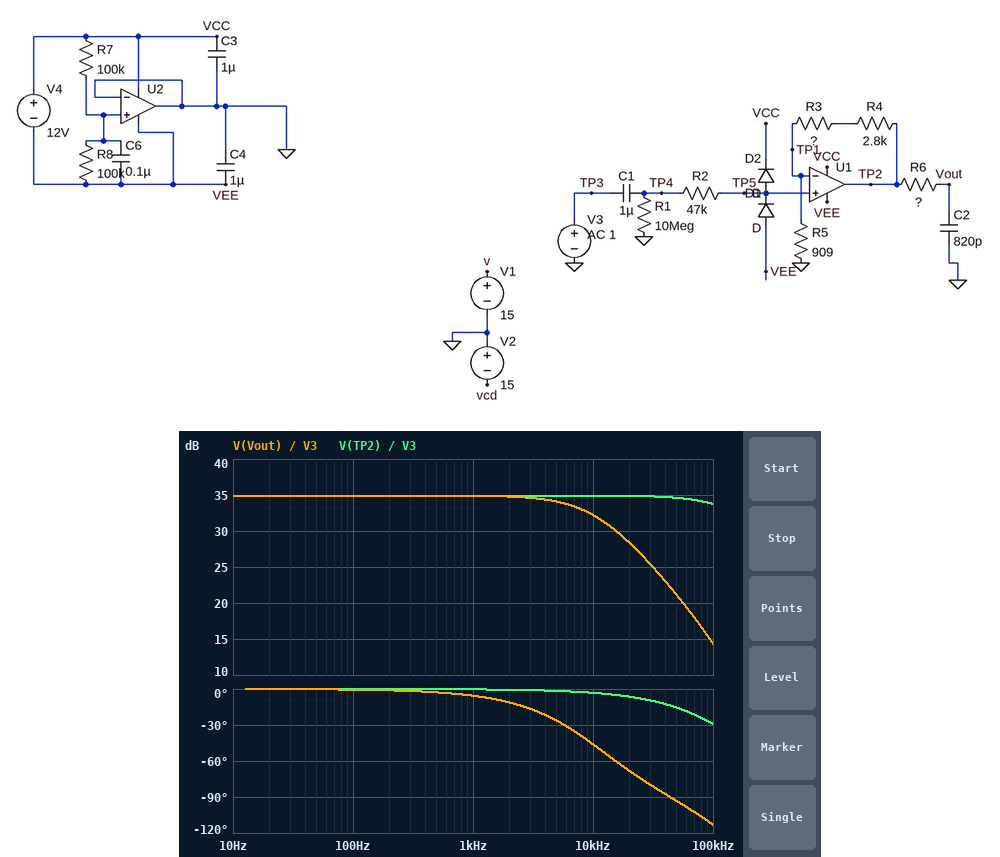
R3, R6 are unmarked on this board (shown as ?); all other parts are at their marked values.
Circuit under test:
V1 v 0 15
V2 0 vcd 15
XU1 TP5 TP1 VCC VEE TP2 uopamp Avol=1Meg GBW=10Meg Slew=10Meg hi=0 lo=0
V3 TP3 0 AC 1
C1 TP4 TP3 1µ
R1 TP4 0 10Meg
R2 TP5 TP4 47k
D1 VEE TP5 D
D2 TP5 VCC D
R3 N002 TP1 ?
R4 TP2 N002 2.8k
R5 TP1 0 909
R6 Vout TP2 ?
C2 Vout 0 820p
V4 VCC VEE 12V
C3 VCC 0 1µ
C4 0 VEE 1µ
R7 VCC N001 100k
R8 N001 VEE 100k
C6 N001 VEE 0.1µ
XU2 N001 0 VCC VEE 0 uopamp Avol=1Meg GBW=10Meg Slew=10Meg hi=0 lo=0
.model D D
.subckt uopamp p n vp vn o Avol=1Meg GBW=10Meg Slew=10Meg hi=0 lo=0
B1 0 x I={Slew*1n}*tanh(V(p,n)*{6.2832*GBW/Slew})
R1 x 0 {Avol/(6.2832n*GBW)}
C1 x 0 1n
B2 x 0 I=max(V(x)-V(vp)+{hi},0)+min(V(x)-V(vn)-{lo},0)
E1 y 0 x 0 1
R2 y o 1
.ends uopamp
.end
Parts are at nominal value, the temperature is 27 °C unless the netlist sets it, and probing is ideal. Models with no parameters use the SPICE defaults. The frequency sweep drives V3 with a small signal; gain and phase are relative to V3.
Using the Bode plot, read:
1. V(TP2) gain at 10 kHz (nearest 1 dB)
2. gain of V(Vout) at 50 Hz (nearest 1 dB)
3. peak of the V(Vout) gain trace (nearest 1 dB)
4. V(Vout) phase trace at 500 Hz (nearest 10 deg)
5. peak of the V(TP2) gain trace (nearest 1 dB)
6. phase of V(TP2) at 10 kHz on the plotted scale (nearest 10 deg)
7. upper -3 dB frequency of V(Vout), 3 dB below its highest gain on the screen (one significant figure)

35 dB
35 dB
35 dB
0 deg
35 dB
0 deg
10 kHz
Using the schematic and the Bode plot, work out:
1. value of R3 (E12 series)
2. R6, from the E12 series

47 kΩ
18 kΩ
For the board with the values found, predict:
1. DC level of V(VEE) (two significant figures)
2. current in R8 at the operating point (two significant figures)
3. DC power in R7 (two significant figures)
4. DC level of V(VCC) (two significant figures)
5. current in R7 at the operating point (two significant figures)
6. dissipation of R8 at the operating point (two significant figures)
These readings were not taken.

-6.0 V
60 µA
360 µW
6.0 V
60 µA
360 µW
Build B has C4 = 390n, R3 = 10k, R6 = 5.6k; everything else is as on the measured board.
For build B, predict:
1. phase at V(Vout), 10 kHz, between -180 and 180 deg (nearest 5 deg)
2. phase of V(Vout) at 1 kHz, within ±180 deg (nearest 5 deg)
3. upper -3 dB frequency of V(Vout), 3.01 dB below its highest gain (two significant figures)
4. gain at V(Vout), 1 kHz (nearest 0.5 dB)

-15 deg
0 deg
35 kHz
23.5 dB
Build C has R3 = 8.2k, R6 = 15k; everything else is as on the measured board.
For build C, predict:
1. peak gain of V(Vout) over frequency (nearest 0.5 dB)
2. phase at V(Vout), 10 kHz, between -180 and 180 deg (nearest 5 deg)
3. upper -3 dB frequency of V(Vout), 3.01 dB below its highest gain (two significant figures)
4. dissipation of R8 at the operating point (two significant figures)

22.5 dB
-40 deg
13 kHz
360 µW
